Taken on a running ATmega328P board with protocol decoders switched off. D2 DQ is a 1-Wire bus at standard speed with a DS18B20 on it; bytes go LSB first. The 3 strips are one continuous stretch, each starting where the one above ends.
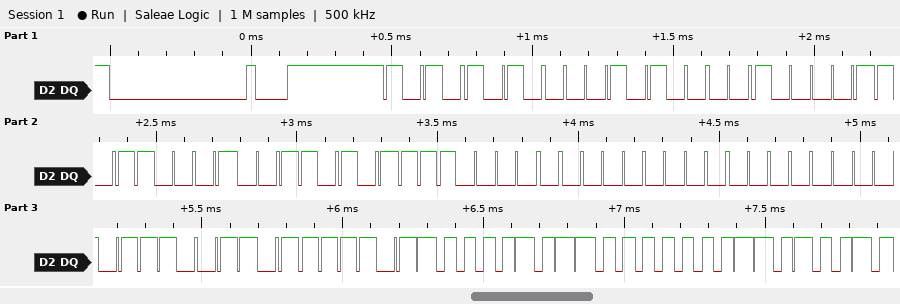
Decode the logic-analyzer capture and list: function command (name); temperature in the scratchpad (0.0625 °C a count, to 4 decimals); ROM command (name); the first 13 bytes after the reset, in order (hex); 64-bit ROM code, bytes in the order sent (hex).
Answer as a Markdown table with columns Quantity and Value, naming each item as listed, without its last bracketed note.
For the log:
| Quantity | Value |
|---|---|
| function command | Read Scratchpad |
| temperature in the scratchpad | 26.0625 °C |
| ROM command | Match ROM |
| the first 13 bytes after the reset, in order | 55 28 84 8D AC 07 00 00 CE BE A1 01 4B |
| 64-bit ROM code, bytes in the order sent | 28 84 8D AC 07 00 00 CE |
